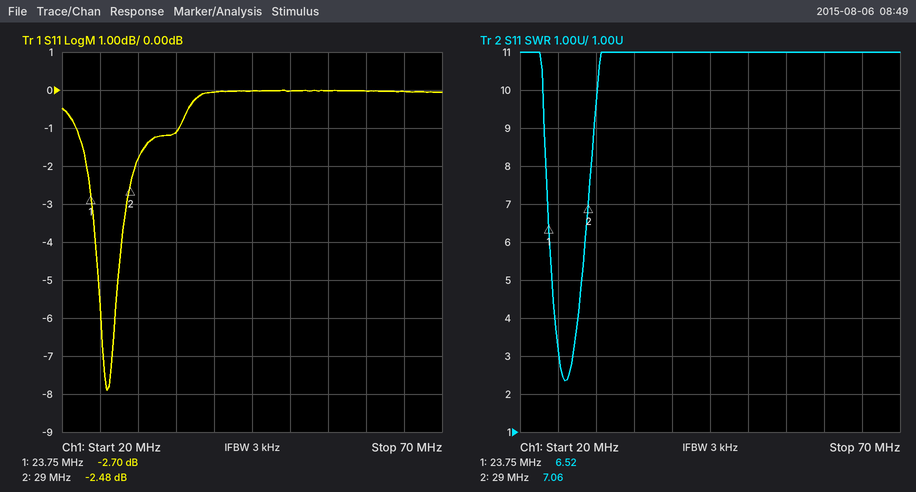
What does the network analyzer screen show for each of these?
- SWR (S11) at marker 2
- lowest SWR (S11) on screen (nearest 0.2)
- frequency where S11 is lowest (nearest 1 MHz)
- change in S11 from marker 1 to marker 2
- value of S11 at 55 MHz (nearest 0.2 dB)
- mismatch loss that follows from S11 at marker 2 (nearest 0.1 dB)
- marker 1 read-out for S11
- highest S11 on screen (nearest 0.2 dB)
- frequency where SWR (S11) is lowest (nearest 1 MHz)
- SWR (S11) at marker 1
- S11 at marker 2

7.06
2.4
26 MHz
0.22 dB
0.0 dB
3.6 dB
-2.70 dB
0.0 dB
26 MHz
6.52
-2.48 dB
